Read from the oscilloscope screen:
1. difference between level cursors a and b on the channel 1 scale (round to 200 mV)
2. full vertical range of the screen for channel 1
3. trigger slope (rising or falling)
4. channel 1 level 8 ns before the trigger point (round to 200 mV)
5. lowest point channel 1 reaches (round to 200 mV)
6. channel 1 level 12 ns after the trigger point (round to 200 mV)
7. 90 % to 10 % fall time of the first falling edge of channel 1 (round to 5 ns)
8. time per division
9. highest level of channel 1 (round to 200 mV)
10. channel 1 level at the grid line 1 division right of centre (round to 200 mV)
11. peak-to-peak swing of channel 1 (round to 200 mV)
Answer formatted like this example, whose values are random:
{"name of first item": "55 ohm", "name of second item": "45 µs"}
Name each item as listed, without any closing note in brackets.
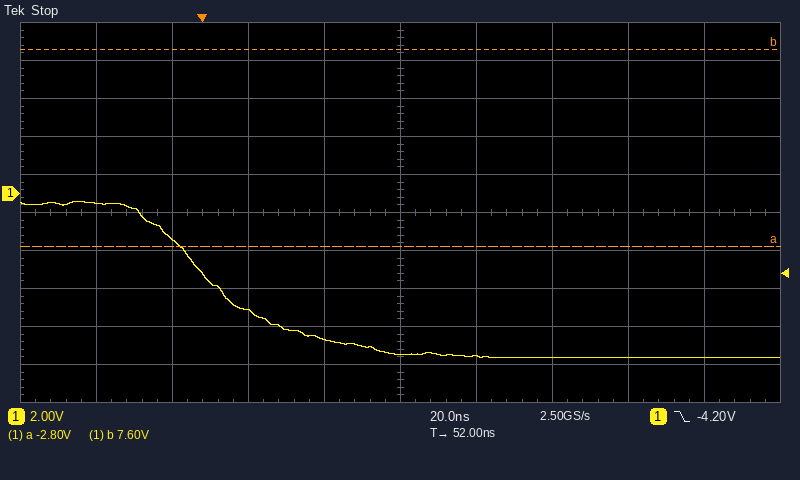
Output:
{"difference between level cursors a and b on the channel 1 scale": "10.4 V", "full vertical range of the screen for channel 1": "20 V", "trigger slope": "falling", "channel 1 level 8 ns before the trigger point": "-2.4 V", "lowest point channel 1 reaches": "-8.6 V", "channel 1 level 12 ns after the trigger point": "-6.2 V", "90 % to 10 % fall time of the first falling edge of channel 1": "50 ns", "time per division": "20 ns", "highest level of channel 1": "-400 mV", "channel 1 level at the grid line 1 division right of centre": "-8.6 V", "peak-to-peak swing of channel 1": "8.2 V"}
